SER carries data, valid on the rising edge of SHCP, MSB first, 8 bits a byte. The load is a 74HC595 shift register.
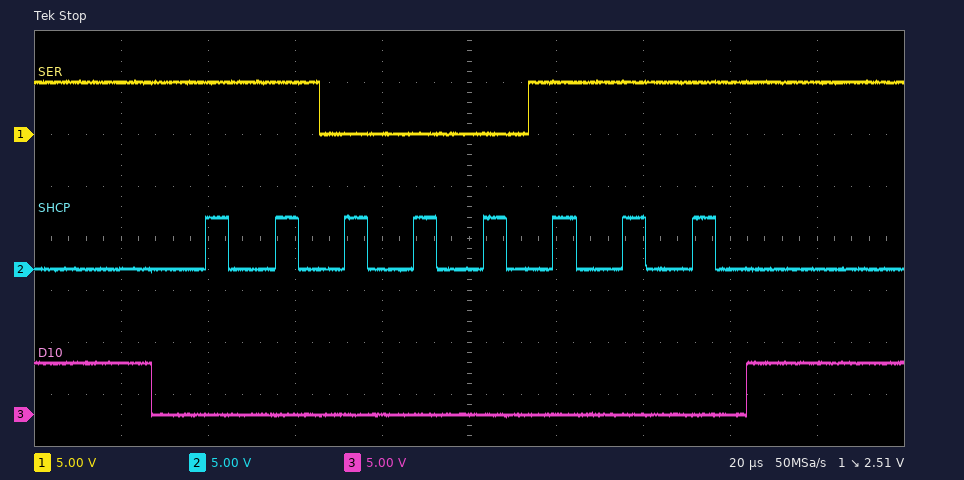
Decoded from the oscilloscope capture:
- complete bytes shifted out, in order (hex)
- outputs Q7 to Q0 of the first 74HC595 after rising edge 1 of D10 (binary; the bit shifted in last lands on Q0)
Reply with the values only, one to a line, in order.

C7
11000111
